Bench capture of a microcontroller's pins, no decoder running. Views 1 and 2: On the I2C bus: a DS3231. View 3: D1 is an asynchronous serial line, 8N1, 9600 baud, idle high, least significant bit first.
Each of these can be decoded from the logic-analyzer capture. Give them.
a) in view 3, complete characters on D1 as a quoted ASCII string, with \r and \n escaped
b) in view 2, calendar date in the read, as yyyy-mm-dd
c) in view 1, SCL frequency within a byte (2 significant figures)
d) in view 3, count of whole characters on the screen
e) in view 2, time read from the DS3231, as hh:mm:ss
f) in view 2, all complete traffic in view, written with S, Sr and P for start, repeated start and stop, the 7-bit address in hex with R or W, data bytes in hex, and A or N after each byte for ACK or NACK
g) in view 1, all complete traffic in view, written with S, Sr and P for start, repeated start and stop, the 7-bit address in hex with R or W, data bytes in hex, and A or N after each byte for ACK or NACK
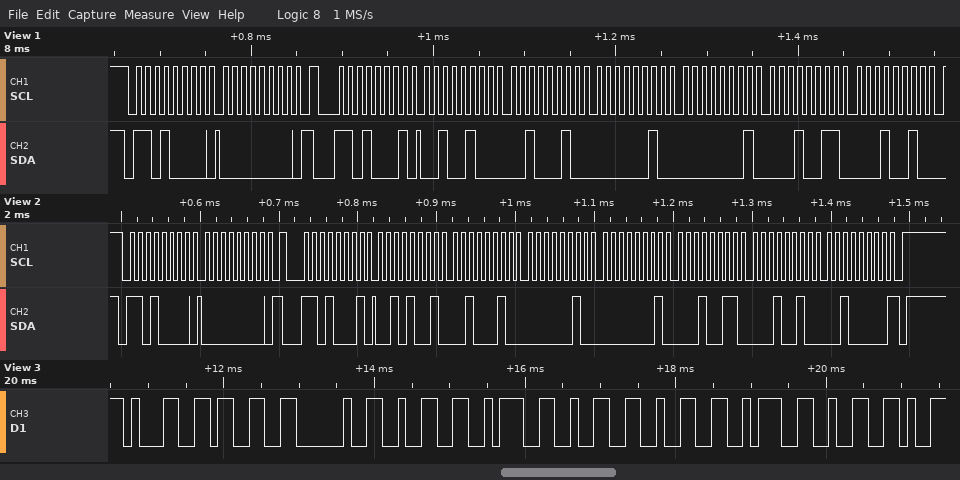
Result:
"13 2:22:2"
2020-12-13
100 kHz
9
02:22:29
S 68W A 00 A Sr 68R A 29 A 22 A 02 A 01 A 13 A 12 A 20 N P
S 68W A 00 A Sr 68R A 24 A 22 A 02 A 01 A 13 A 12 A
